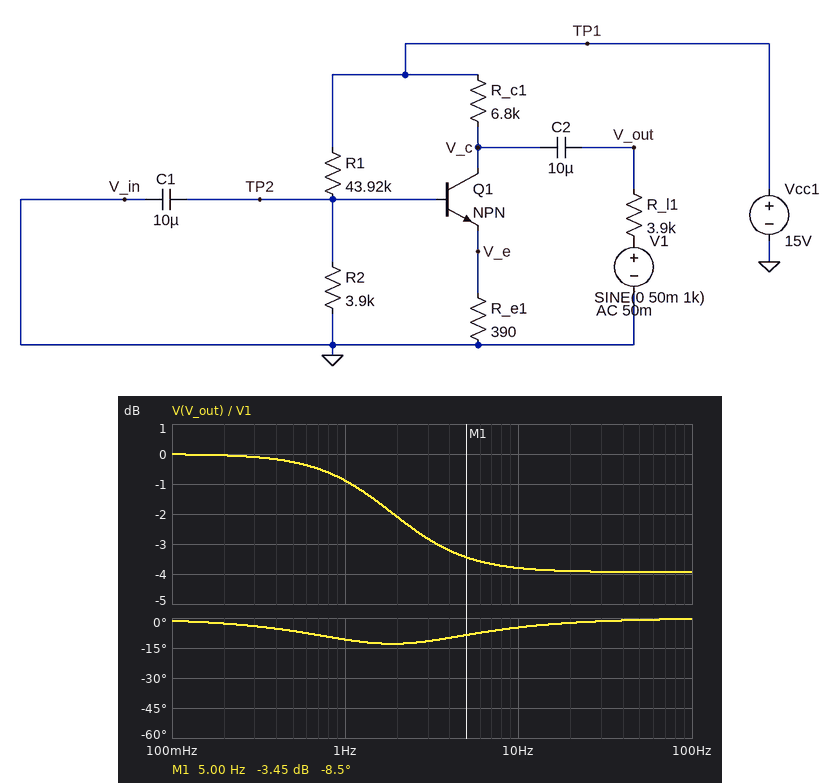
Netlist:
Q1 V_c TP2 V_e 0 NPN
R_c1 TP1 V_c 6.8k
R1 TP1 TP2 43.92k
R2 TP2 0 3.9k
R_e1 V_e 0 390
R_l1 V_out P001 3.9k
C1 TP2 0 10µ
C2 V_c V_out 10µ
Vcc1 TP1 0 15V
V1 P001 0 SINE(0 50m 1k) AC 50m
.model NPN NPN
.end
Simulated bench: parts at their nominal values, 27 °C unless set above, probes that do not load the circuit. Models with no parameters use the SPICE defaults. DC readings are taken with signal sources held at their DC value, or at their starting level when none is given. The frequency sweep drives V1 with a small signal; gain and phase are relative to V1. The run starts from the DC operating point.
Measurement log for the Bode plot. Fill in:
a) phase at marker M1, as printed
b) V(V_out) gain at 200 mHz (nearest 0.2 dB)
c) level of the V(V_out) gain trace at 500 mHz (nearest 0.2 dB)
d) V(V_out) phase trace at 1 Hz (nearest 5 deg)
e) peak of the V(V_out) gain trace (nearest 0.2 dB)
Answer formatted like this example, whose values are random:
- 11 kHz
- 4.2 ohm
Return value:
- -8.5 deg
- 0 dB
- -0.2 dB
- -10 deg
- 0 dB
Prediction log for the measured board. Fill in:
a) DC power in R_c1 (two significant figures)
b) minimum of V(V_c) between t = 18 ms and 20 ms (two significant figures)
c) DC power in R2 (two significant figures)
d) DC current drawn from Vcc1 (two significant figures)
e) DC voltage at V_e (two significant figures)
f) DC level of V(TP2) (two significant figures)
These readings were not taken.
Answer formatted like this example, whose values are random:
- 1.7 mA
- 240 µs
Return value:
- 7.4 mW
- 7.9 V
- 360 µW
- 1.4 mA
- 410 mV
- 1.2 V
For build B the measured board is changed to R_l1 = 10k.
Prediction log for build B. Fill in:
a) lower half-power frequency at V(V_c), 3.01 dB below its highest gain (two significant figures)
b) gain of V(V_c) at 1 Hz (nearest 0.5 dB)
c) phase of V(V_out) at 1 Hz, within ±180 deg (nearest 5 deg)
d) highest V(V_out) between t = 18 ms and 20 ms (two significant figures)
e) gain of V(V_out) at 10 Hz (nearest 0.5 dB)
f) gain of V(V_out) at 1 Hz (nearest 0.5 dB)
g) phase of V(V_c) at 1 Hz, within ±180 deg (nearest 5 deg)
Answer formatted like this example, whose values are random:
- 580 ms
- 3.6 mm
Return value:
- 950 mHz
- -10.5 dB
- -25 deg
- 20 mV
- -7.5 dB
- -2.5 dB
- 45 deg
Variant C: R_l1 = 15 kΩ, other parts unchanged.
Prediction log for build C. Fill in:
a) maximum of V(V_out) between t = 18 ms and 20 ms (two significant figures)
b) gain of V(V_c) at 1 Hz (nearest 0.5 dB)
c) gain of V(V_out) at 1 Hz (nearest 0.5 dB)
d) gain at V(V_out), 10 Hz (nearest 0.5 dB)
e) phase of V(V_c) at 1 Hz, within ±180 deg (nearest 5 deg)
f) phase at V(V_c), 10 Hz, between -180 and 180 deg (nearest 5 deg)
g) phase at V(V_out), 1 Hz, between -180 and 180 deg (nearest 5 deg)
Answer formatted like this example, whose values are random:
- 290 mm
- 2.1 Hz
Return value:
- 16 mV
- -12.0 dB
- -4.0 dB
- -10.0 dB
- 35 deg
- 5 deg
- -30 deg
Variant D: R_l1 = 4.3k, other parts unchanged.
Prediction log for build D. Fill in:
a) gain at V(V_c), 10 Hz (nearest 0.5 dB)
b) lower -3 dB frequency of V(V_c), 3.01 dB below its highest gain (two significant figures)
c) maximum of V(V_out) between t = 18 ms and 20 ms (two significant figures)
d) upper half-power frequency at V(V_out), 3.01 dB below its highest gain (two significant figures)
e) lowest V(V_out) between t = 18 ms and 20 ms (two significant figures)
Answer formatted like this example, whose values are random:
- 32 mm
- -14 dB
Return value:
- -4.5 dB
- 1.4 Hz
- 31 mV
- 2.9 Hz
- -31 mV
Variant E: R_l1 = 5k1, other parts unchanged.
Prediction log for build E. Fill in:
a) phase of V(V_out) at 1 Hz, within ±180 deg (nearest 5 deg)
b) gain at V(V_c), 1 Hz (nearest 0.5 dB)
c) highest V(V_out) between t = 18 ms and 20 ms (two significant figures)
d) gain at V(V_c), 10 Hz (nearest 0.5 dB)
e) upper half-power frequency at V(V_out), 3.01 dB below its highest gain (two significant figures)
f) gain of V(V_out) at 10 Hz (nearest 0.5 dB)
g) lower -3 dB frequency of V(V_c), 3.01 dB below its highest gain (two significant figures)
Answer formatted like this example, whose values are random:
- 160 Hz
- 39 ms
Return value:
- -15 deg
- -9.5 dB
- 29 mV
- -5.0 dB
- 2.3 Hz
- -4.5 dB
- 1.3 Hz
